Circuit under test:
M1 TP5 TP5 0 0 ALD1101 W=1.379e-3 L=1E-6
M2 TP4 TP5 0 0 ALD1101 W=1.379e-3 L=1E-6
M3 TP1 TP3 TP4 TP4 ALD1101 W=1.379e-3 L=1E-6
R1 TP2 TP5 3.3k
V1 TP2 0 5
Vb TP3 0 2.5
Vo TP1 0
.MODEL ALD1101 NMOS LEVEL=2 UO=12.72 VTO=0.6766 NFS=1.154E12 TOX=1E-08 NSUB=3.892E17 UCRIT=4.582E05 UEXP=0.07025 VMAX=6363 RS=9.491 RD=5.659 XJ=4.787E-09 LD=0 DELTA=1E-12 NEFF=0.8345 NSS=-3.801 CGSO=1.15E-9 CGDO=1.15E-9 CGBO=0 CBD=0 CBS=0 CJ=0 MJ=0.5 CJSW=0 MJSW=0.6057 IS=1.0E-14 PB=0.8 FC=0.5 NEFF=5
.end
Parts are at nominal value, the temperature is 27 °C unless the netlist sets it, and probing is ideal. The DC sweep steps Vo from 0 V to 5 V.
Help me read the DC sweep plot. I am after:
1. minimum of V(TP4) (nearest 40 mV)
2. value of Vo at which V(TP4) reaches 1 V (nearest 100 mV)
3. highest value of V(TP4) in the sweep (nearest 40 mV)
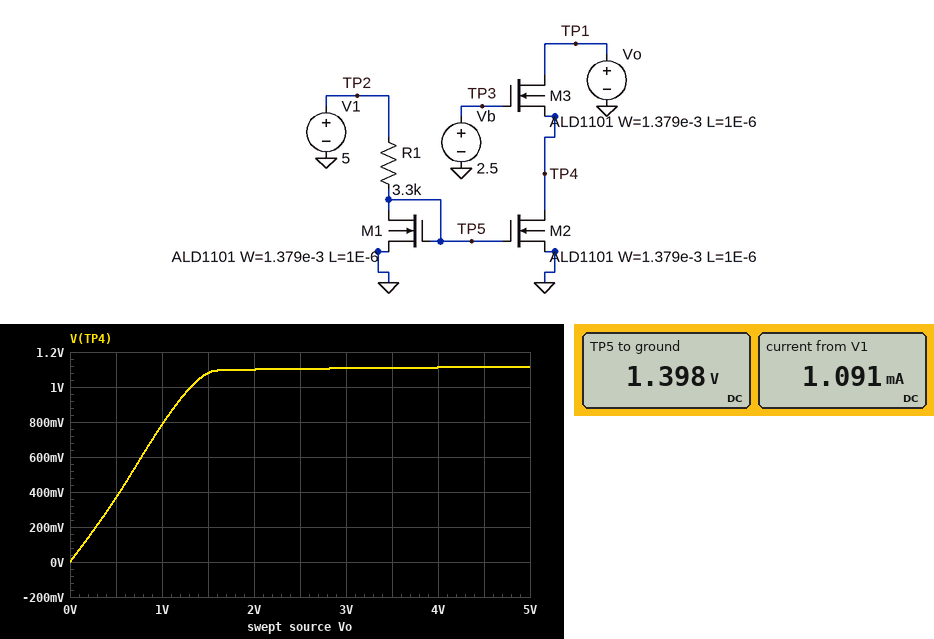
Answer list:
0 V
1.3 V
1.12 V
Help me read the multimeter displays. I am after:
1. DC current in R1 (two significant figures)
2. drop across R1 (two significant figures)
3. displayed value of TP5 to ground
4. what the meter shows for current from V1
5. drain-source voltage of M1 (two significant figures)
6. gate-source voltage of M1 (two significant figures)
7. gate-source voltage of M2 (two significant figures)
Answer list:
1.1 mA
3.6 V
1.398 V
1.091 mA
1.4 V
1.4 V
1.4 V
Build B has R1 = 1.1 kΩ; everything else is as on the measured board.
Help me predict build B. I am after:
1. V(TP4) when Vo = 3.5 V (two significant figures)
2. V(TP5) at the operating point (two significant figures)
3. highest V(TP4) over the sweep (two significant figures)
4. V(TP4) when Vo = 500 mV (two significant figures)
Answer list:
680 mV
1.9 V
690 mV
290 mV
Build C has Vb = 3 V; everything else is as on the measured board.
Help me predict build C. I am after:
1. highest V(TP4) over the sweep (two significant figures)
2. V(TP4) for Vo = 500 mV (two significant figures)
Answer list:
1.6 V
390 mV
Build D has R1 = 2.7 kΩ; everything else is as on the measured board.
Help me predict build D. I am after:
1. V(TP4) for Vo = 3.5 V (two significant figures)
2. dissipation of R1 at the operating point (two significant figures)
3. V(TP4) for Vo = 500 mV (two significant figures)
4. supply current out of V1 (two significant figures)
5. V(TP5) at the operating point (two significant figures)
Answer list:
1.0 V
4.6 mW
350 mV
1.3 mA
1.5 V
